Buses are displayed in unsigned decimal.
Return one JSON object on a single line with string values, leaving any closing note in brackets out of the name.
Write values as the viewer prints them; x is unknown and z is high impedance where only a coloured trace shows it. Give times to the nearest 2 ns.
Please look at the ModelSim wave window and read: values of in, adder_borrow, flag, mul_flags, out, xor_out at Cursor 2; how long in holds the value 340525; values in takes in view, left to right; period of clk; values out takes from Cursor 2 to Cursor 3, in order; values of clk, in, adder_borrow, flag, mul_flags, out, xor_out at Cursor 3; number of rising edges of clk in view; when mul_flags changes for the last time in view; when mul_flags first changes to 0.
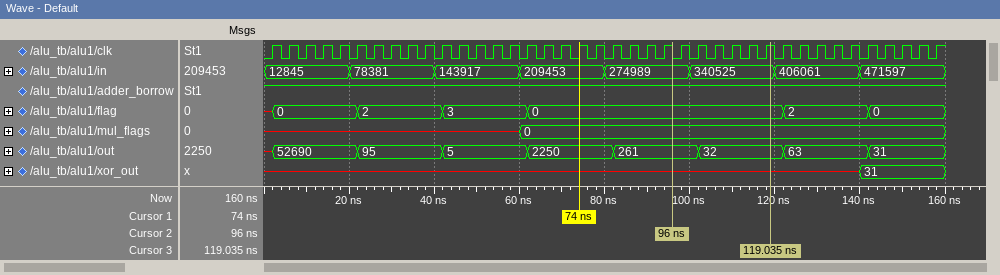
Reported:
{"values of in, adder_borrow, flag, mul_flags, out, xor_out at Cursor 2": "in=274989, adder_borrow=1, flag=0, mul_flags=0, out=261, xor_out=x", "how long in holds the value 340525": "20 ns", "values in takes in view, left to right": "12845, 78381, 143917, 209453, 274989, 340525, 406061, 471597", "period of clk": "4 ns", "values out takes from Cursor 2 to Cursor 3, in order": "261, 32", "values of clk, in, adder_borrow, flag, mul_flags, out, xor_out at Cursor 3": "clk=1, in=340525, adder_borrow=1, flag=0, mul_flags=0, out=32, xor_out=x", "number of rising edges of clk in view": "40", "when mul_flags changes for the last time in view": "60 ns", "when mul_flags first changes to 0": "60 ns"}
